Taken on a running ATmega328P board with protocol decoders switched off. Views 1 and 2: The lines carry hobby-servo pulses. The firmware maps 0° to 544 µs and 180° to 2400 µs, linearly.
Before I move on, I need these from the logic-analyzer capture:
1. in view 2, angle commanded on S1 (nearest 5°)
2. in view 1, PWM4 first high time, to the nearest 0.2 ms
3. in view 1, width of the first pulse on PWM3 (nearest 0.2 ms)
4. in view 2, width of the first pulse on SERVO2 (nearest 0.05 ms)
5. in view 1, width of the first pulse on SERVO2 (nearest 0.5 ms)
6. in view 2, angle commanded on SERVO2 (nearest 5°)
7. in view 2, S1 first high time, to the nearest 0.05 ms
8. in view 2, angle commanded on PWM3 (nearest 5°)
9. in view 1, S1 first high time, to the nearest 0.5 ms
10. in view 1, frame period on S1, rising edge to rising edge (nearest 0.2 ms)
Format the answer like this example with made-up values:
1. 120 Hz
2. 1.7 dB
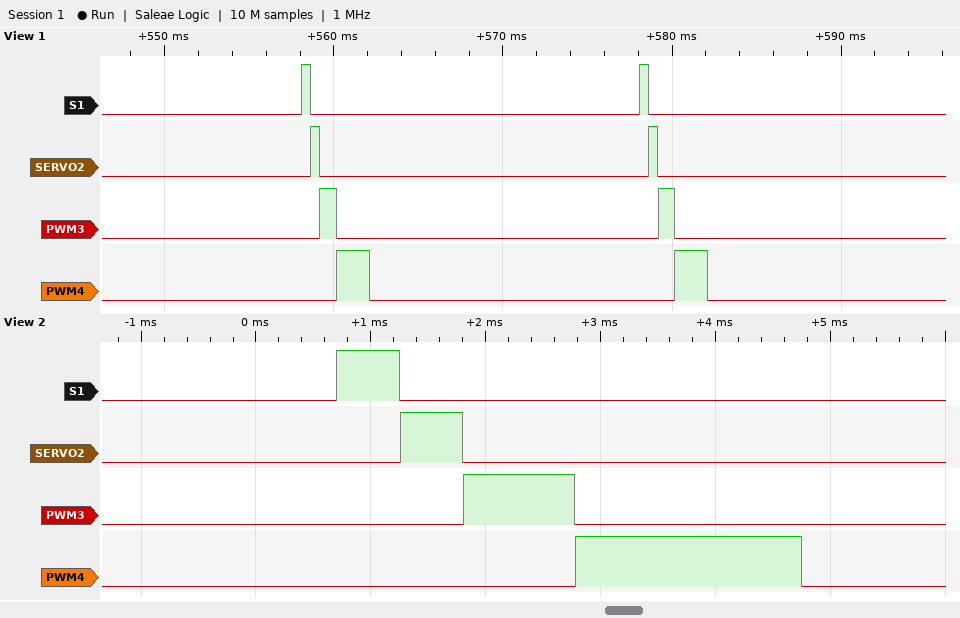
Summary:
1. 0°
2. 2.0 ms
3. 1.0 ms
4. 0.55 ms
5. 0.5 ms
6. 0°
7. 0.55 ms
8. 40°
9. 0.5 ms
10. 20.0 ms
